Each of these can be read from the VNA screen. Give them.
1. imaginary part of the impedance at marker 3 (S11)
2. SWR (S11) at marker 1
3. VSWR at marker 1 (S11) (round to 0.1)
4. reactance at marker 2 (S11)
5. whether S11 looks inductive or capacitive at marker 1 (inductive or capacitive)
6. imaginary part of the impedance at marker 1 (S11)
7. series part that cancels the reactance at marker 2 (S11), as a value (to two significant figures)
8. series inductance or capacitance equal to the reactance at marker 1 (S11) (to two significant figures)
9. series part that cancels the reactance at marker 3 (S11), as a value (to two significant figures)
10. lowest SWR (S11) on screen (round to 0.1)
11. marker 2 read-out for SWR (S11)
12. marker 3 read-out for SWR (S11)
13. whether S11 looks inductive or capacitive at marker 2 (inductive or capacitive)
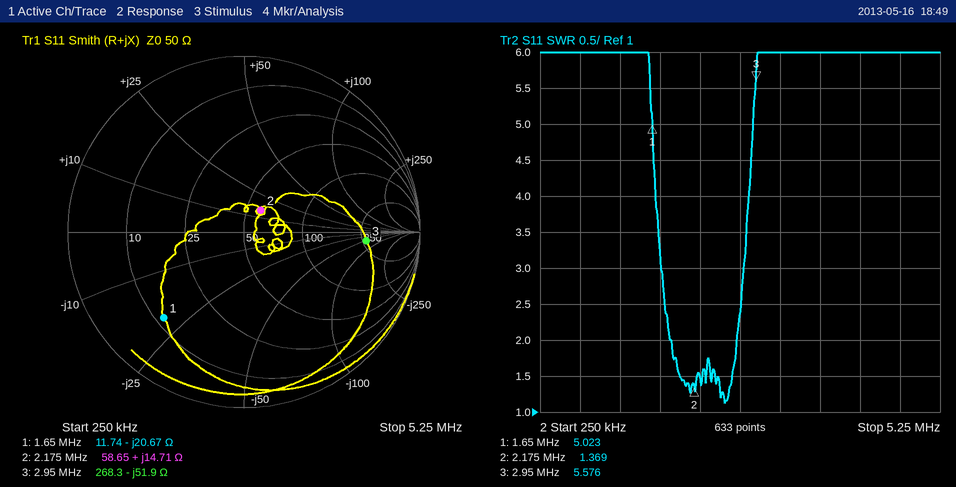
-51.9 Ω
5.023
5.0
+14.71 Ω
capacitive
-20.67 Ω
5.0 nF
4.7 nF
2.8 µH
1.1
1.369
5.576
inductive
